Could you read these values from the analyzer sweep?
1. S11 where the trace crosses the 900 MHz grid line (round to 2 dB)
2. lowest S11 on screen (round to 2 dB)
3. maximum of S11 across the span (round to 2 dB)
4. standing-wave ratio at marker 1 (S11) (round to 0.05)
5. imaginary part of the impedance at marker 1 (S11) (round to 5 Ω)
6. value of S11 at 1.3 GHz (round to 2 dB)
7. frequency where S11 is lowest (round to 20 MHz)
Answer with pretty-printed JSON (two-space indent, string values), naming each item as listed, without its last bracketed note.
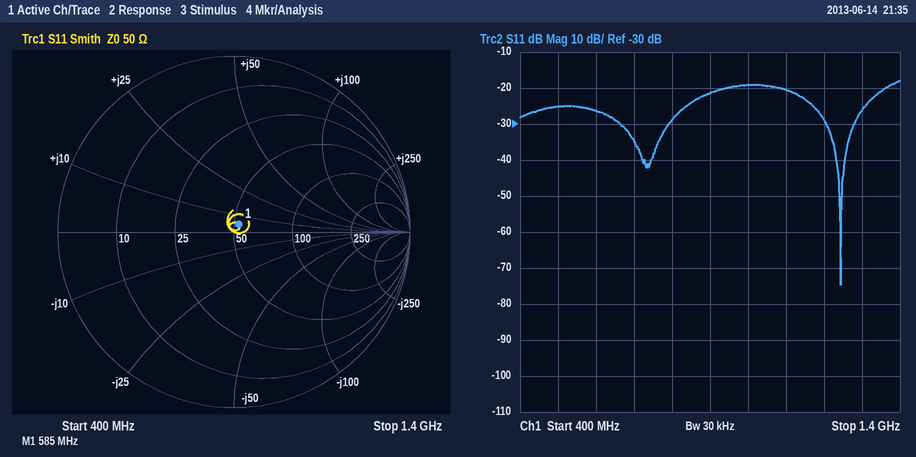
{
  "S11 where the trace crosses the 900 MHz grid line": "-22 dB",
  "lowest S11 on screen": "-74 dB",
  "maximum of S11 across the span": "-18 dB",
  "standing-wave ratio at marker 1 (S11)": "1.10",
  "imaginary part of the impedance at marker 1 (S11)": "+5 Ω",
  "value of S11 at 1.3 GHz": "-26 dB",
  "frequency where S11 is lowest": "1.24 GHz"
}
